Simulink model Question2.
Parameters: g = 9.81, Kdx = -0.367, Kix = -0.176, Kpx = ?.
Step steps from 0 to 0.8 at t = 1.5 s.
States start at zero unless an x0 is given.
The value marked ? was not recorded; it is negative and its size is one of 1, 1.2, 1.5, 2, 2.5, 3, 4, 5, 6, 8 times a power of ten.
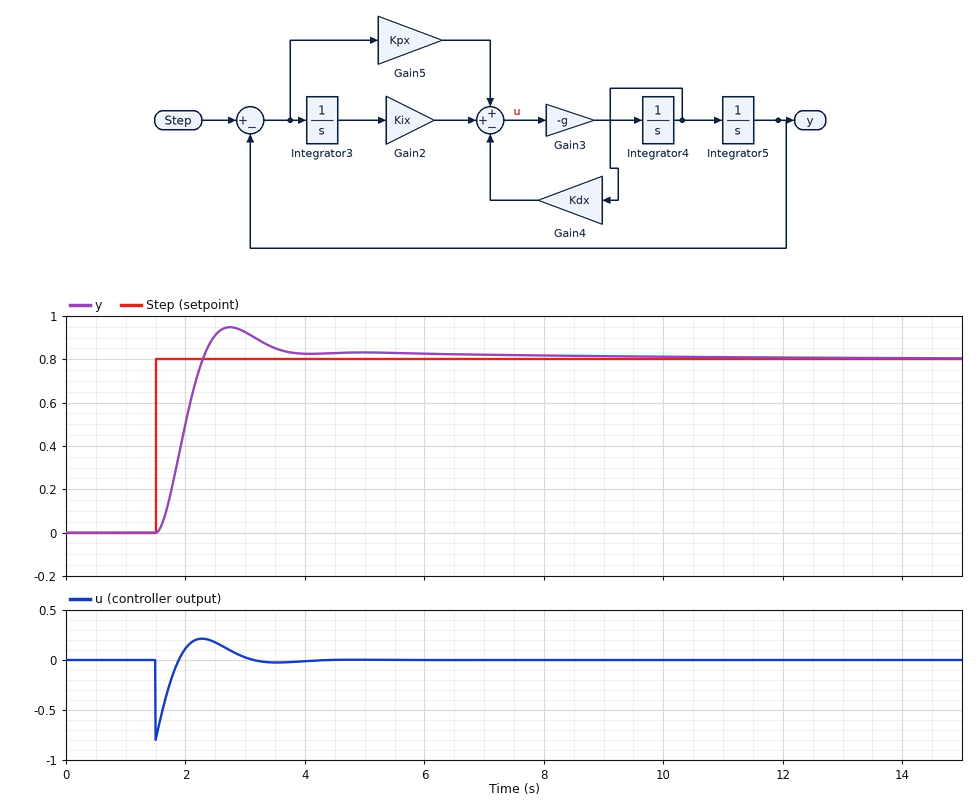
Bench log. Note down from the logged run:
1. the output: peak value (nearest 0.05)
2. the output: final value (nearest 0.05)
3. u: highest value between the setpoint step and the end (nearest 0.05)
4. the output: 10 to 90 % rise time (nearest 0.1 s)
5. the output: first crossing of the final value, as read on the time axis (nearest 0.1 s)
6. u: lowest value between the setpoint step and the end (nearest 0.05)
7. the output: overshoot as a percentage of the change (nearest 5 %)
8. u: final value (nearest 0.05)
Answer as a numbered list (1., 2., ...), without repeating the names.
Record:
1. 0.95
2. 0.80
3. 0.20
4. 0.5 s
5. 2.3 s
6. -0.80
7. 20 %
8. 0.00
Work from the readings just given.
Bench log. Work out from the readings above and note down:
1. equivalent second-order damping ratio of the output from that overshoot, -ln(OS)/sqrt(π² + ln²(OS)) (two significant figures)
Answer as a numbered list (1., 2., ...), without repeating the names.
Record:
1. 0.46
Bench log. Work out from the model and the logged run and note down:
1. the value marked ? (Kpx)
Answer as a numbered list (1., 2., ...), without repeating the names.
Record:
1. -1
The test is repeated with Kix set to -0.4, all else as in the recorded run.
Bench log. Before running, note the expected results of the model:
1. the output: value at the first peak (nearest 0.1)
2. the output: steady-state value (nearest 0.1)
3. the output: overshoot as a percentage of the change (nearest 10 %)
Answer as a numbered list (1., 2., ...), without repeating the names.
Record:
1. 1.0
2. 0.8
3. 30 %
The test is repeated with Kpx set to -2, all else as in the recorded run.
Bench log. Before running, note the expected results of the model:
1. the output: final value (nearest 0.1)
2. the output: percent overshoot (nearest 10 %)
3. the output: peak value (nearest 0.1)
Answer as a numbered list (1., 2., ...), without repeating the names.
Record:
1. 0.8
2. 30 %
3. 1.0
